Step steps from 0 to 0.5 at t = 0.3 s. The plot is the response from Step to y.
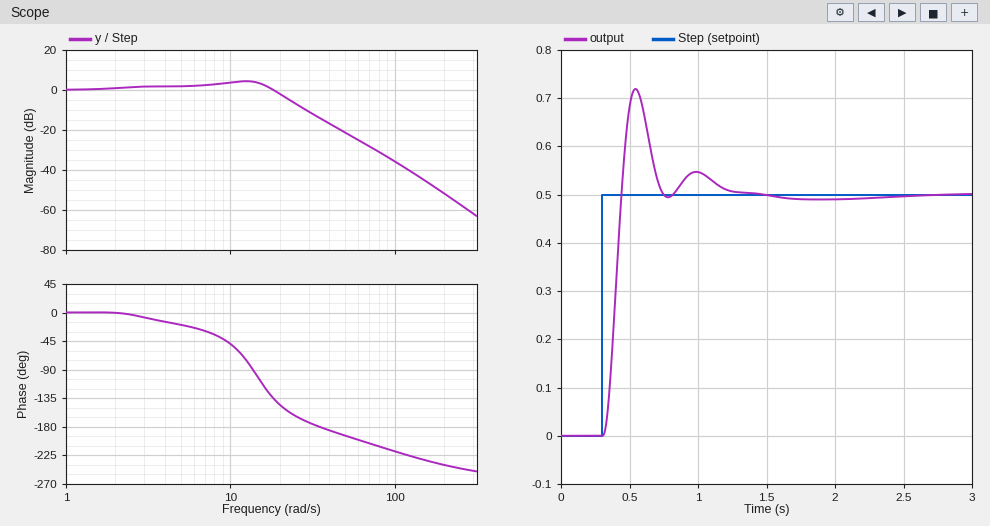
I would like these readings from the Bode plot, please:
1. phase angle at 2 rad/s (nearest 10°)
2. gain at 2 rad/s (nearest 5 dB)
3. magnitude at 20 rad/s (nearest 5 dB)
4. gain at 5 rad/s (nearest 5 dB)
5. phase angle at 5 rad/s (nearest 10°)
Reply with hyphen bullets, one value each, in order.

- 0°
- 0 dB
- 0 dB
- 0 dB
- -20°
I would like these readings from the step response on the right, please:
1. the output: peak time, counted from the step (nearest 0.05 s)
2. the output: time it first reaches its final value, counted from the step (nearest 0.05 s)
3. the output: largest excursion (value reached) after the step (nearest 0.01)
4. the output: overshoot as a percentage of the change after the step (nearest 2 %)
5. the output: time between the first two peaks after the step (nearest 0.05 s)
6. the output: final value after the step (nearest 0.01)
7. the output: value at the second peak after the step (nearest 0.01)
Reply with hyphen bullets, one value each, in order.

- 0.25 s
- 0.15 s
- 0.72
- 44 %
- 0.45 s
- 0.50
- 0.55
